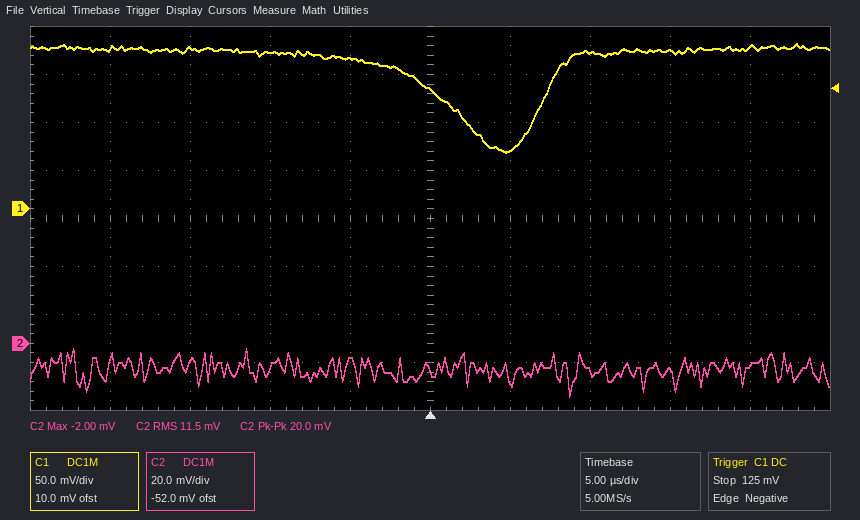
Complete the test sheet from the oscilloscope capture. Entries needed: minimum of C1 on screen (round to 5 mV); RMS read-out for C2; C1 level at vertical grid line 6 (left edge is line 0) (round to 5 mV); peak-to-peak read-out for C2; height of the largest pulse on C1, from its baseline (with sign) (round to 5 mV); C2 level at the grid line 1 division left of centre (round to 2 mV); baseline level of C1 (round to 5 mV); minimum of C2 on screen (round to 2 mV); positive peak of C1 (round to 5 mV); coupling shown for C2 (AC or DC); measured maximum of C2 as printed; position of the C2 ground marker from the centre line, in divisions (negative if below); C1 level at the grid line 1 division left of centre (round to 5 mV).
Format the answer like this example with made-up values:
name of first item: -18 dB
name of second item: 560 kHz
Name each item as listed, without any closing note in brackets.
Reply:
minimum of C1 on screen: 60 mV
RMS read-out for C2: 11.5 mV
C1 level at vertical grid line 6 (left edge is line 0): 60 mV
peak-to-peak read-out for C2: 20.0 mV
height of the largest pulse on C1, from its baseline (with sign): -105 mV
C2 level at the grid line 1 division left of centre: -8 mV
baseline level of C1: 165 mV
minimum of C2 on screen: -22 mV
positive peak of C1: 170 mV
coupling shown for C2: DC
measured maximum of C2 as printed: -2.00 mV
position of the C2 ground marker from the centre line, in divisions: -2.6 div
C1 level at the grid line 1 division left of centre: 155 mV
